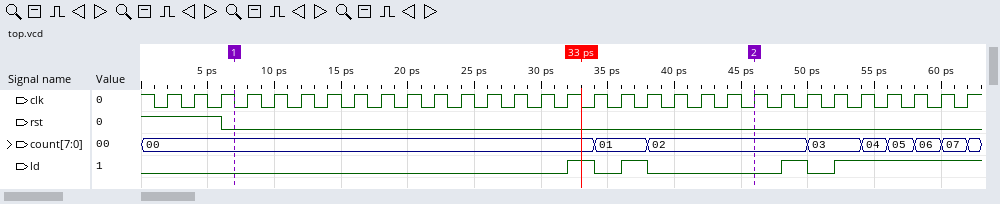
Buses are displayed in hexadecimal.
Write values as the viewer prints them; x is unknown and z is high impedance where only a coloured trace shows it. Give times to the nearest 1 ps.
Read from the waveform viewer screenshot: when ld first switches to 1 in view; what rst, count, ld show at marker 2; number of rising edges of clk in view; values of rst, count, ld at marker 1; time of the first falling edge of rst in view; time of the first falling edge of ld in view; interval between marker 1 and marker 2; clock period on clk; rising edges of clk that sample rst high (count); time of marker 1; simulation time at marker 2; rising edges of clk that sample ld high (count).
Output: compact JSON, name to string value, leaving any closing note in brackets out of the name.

{"when ld first switches to 1 in view": "32 ps", "what rst, count, ld show at marker 2": "rst=0, count=02, ld=0", "number of rising edges of clk in view": "31", "values of rst, count, ld at marker 1": "rst=0, count=00, ld=0", "time of the first falling edge of rst in view": "6 ps", "time of the first falling edge of ld in view": "34 ps", "interval between marker 1 and marker 2": "39 ps", "clock period on clk": "2 ps", "rising edges of clk that sample rst high": "3", "time of marker 1": "7 ps", "simulation time at marker 2": "46 ps", "rising edges of clk that sample ld high": "8"}
